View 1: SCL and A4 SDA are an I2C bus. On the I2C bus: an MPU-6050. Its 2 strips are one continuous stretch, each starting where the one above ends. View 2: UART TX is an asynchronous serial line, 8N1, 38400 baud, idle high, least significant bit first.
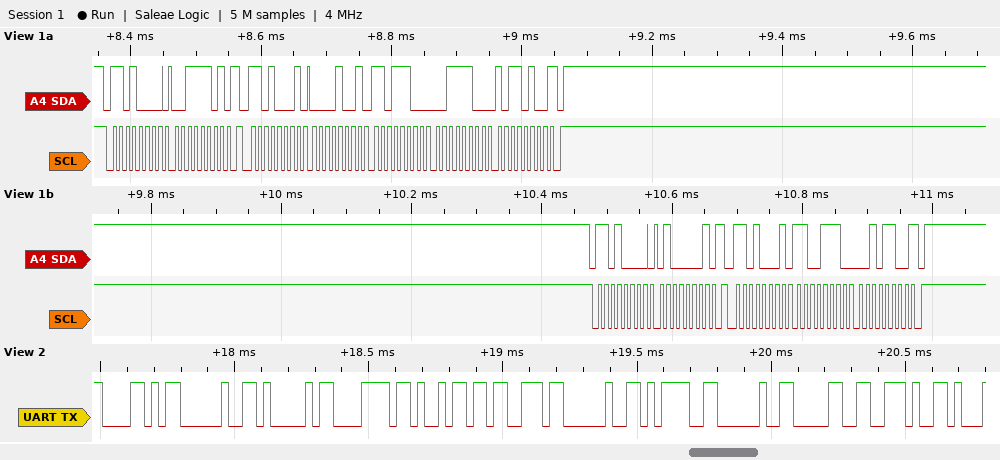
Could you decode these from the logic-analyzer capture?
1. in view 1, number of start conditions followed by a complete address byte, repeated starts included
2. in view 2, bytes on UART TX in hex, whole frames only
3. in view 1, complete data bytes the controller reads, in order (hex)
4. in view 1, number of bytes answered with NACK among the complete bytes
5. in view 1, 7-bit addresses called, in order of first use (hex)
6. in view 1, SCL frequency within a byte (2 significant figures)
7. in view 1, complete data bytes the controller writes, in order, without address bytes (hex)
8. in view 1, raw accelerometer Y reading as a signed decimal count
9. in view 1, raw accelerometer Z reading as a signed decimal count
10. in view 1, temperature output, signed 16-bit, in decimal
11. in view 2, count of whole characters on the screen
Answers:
4
58 20 41 78 69 73 20 3D 20 30 2E
09 DC 3C B4 CE 2C
2
0x68
100 kHz
3D 41
2524
15540
-12756
11
